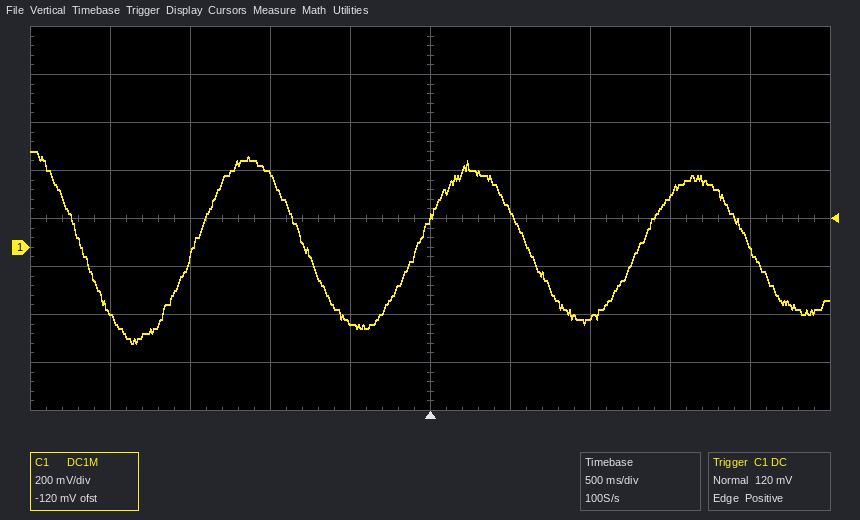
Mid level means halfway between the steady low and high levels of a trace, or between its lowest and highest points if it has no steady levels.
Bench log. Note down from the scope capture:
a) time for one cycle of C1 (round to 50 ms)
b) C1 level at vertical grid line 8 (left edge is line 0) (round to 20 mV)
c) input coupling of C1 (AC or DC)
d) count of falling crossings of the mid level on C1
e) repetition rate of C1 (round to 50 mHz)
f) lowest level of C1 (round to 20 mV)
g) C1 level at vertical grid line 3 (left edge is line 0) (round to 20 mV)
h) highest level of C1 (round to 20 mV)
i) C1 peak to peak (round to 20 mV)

1.40 s
220 mV
DC
4
700 mHz
-400 mV
300 mV
400 mV
800 mV
